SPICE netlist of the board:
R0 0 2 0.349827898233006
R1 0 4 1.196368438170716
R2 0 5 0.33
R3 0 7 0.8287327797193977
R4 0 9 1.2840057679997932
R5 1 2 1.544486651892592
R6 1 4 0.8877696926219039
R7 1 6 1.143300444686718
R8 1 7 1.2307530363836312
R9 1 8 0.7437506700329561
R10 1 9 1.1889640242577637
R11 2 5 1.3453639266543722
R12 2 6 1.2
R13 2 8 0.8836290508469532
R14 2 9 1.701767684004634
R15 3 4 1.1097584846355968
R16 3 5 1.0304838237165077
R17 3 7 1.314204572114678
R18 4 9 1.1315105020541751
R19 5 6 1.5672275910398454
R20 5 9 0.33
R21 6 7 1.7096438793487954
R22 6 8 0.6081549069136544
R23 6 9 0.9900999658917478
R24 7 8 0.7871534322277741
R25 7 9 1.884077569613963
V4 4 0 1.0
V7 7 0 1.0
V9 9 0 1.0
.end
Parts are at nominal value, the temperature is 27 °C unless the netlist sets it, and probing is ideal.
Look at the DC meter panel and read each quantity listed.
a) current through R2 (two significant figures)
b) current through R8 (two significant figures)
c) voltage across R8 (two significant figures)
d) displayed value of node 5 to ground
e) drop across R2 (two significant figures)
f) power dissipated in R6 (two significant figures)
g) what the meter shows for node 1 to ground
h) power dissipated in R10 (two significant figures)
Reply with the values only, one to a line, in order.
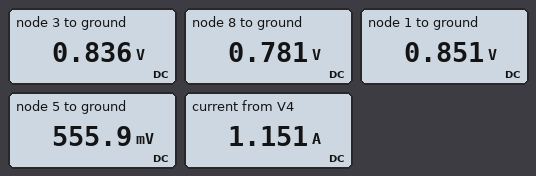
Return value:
1.7 A
120 mA
150 mV
555.9 mV
560 mV
25 mW
0.851 V
19 mW
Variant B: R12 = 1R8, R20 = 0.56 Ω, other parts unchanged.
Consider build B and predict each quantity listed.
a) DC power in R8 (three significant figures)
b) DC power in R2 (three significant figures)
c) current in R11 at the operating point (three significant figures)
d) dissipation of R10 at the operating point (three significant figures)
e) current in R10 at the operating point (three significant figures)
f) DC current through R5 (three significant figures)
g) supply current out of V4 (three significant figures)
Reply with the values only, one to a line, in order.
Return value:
18.9 mW
676 mW
32.1 mA
19.6 mW
128 mA
271 mA
1.18 A
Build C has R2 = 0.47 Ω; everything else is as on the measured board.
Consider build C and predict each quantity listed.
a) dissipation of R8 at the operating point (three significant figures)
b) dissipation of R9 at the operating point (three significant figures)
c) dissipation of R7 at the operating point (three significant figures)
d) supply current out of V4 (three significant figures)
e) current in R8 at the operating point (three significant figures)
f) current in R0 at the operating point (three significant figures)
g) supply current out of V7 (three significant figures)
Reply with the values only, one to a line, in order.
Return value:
16.8 mW
6.14 mW
3.50 mW
1.12 A
117 mA
1.33 A
1.82 A
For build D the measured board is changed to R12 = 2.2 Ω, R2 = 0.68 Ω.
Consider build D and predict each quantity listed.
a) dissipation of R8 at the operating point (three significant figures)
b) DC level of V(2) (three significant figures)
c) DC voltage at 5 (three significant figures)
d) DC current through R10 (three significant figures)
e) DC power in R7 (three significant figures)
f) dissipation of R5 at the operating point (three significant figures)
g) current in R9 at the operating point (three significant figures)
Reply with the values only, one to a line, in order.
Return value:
15.0 mW
459 mV
695 mV
114 mA
1.04 mW
106 mW
85.5 mA
